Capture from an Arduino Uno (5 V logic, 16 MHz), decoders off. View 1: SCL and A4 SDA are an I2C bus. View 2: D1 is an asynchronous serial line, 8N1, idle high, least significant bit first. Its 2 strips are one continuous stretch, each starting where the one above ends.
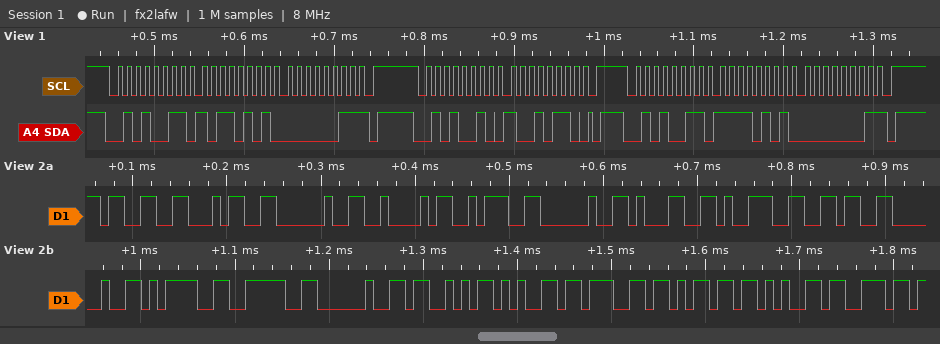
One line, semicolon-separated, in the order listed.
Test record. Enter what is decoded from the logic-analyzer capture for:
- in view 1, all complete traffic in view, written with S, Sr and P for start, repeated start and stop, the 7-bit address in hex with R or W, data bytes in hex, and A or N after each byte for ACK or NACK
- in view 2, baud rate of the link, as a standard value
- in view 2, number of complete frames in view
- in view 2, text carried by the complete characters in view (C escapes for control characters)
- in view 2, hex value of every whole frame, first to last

S 29R A B5 A 03 N P S 29W A 96 A P S 29R A F5 A 01 N P; 115200 baud; 19; "34 B: 196 => Segmen"; 33 34 20 42 3A 20 31 39 36 20 3D 3E 20 53 65 67 6D 65 6E
